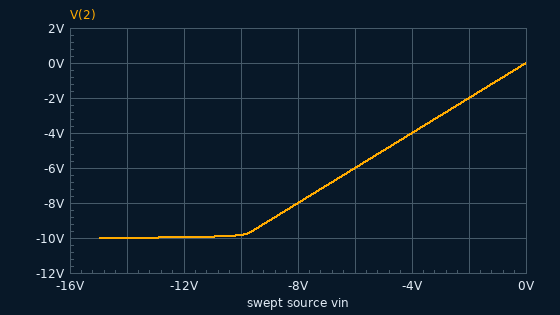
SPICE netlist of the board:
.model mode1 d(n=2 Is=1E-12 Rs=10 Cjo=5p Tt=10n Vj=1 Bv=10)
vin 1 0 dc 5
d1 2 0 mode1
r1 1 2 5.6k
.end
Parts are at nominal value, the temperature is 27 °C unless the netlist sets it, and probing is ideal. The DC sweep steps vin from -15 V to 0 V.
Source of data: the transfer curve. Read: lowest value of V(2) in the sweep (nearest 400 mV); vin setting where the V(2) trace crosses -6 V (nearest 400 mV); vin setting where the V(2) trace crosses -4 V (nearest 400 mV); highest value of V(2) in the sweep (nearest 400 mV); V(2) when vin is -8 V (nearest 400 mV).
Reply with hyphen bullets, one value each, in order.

- -10.0 V
- -6.0 V
- -4.0 V
- 0 V
- -8.0 V
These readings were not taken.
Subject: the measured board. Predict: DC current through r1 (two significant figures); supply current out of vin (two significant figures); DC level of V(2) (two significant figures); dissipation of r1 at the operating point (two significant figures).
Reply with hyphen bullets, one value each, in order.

- 700 µA
- 700 µA
- 1.1 V
- 2.8 mW
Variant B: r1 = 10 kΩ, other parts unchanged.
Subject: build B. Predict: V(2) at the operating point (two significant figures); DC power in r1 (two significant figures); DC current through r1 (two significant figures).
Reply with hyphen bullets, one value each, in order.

- 1.0 V
- 1.6 mW
- 400 µA
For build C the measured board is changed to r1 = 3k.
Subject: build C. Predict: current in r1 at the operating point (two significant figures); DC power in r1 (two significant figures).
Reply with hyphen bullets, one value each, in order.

- 1.3 mA
- 5.1 mW
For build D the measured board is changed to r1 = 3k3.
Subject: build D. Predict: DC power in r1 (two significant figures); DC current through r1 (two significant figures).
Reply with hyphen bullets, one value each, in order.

- 4.6 mW
- 1.2 mA
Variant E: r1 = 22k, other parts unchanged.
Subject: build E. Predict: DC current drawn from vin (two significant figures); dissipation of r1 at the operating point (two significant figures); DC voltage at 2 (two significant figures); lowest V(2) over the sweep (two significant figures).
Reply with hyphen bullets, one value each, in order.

- 180 µA
- 730 µW
- 990 mV
- -9.9 V
